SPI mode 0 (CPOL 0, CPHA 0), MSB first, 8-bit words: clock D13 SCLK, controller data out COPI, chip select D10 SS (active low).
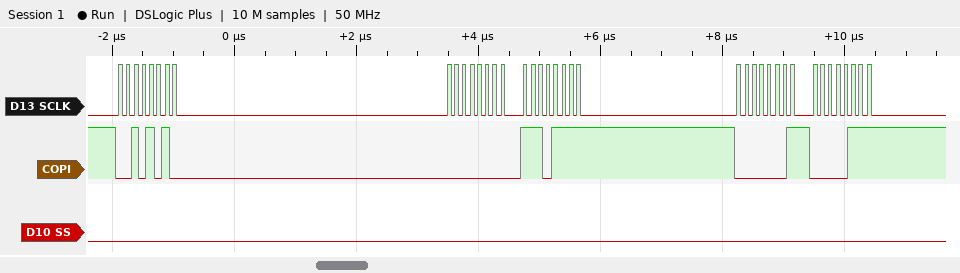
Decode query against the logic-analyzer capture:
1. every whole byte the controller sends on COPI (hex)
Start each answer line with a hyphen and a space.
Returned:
- 2A 00 EF 01 07
